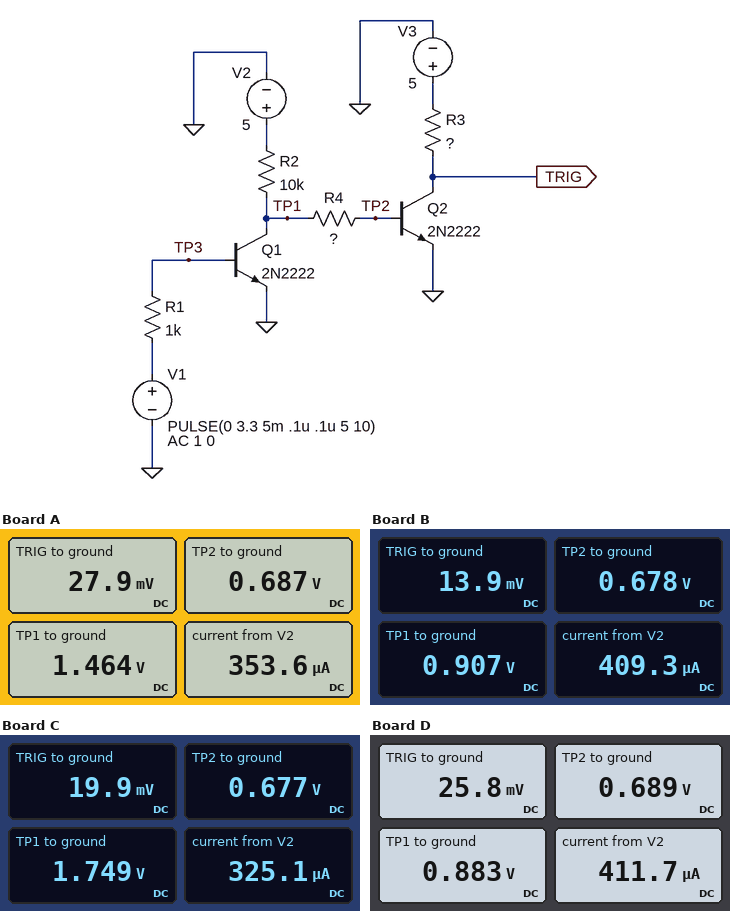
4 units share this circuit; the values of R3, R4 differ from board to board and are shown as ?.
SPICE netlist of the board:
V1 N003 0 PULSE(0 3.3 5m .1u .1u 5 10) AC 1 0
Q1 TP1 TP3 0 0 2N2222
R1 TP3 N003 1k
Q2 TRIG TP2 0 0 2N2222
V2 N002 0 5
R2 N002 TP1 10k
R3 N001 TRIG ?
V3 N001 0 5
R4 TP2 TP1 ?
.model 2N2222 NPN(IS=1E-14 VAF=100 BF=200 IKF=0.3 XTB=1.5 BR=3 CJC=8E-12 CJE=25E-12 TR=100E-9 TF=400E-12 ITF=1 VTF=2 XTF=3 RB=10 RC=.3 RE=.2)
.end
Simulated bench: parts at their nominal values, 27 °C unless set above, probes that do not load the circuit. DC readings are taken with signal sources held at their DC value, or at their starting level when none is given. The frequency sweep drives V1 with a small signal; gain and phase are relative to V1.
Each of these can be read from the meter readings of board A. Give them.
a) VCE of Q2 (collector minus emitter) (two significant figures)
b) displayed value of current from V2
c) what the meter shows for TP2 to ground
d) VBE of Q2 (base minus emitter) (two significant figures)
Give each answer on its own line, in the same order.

28 mV
353.6 µA
0.687 V
690 mV
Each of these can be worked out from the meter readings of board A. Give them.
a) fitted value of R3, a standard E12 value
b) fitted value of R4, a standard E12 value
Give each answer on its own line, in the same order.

3.3 kΩ
2.2 kΩ
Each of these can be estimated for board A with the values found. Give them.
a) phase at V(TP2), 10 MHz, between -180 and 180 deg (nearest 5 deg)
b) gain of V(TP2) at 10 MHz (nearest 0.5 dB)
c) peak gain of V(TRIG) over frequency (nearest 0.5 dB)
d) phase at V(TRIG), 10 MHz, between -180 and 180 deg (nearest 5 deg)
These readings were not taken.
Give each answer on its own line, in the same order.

-5 deg
-53.5 dB
-59.5 dB
15 deg
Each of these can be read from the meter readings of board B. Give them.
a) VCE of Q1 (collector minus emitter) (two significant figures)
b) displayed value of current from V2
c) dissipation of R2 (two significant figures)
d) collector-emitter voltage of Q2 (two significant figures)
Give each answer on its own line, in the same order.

910 mV
409.3 µA
1.7 mW
14 mV
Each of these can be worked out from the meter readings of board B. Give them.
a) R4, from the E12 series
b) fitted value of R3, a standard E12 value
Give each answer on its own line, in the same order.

560 Ω
12 kΩ
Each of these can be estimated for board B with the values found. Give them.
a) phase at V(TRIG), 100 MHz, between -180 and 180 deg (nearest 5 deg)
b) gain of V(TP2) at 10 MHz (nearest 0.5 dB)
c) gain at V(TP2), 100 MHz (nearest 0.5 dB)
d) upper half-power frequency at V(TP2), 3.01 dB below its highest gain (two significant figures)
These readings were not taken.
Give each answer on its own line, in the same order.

-85 deg
-48.5 dB
-54.5 dB
63 MHz
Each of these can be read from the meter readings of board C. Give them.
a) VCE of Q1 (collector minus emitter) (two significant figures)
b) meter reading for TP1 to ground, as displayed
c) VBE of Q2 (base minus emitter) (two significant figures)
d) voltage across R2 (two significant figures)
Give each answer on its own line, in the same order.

1.7 V
1.749 V
680 mV
3.3 V
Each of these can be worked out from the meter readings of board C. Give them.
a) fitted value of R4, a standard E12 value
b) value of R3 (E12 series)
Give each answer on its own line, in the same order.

3.3 kΩ
6.8 kΩ
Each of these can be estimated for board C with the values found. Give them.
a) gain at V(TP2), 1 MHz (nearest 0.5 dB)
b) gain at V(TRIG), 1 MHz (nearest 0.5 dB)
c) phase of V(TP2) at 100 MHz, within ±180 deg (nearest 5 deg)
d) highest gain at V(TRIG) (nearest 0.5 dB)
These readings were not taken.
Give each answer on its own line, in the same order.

-61.0 dB
-67.0 dB
-95 deg
-58.5 dB
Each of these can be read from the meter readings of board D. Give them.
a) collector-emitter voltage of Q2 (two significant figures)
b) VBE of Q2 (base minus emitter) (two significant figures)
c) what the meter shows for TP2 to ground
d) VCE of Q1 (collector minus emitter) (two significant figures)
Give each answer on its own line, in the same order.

26 mV
690 mV
0.689 V
880 mV
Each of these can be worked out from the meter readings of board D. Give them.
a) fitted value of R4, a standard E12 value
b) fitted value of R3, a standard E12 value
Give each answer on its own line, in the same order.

470 Ω
3.3 kΩ
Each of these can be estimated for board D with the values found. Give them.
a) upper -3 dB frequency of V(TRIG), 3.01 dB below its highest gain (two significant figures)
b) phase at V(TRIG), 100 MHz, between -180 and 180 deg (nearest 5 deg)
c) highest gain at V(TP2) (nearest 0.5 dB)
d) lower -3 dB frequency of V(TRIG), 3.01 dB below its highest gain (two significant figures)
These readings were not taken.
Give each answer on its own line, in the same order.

72 MHz
-75 deg
-50.0 dB
3.6 MHz
